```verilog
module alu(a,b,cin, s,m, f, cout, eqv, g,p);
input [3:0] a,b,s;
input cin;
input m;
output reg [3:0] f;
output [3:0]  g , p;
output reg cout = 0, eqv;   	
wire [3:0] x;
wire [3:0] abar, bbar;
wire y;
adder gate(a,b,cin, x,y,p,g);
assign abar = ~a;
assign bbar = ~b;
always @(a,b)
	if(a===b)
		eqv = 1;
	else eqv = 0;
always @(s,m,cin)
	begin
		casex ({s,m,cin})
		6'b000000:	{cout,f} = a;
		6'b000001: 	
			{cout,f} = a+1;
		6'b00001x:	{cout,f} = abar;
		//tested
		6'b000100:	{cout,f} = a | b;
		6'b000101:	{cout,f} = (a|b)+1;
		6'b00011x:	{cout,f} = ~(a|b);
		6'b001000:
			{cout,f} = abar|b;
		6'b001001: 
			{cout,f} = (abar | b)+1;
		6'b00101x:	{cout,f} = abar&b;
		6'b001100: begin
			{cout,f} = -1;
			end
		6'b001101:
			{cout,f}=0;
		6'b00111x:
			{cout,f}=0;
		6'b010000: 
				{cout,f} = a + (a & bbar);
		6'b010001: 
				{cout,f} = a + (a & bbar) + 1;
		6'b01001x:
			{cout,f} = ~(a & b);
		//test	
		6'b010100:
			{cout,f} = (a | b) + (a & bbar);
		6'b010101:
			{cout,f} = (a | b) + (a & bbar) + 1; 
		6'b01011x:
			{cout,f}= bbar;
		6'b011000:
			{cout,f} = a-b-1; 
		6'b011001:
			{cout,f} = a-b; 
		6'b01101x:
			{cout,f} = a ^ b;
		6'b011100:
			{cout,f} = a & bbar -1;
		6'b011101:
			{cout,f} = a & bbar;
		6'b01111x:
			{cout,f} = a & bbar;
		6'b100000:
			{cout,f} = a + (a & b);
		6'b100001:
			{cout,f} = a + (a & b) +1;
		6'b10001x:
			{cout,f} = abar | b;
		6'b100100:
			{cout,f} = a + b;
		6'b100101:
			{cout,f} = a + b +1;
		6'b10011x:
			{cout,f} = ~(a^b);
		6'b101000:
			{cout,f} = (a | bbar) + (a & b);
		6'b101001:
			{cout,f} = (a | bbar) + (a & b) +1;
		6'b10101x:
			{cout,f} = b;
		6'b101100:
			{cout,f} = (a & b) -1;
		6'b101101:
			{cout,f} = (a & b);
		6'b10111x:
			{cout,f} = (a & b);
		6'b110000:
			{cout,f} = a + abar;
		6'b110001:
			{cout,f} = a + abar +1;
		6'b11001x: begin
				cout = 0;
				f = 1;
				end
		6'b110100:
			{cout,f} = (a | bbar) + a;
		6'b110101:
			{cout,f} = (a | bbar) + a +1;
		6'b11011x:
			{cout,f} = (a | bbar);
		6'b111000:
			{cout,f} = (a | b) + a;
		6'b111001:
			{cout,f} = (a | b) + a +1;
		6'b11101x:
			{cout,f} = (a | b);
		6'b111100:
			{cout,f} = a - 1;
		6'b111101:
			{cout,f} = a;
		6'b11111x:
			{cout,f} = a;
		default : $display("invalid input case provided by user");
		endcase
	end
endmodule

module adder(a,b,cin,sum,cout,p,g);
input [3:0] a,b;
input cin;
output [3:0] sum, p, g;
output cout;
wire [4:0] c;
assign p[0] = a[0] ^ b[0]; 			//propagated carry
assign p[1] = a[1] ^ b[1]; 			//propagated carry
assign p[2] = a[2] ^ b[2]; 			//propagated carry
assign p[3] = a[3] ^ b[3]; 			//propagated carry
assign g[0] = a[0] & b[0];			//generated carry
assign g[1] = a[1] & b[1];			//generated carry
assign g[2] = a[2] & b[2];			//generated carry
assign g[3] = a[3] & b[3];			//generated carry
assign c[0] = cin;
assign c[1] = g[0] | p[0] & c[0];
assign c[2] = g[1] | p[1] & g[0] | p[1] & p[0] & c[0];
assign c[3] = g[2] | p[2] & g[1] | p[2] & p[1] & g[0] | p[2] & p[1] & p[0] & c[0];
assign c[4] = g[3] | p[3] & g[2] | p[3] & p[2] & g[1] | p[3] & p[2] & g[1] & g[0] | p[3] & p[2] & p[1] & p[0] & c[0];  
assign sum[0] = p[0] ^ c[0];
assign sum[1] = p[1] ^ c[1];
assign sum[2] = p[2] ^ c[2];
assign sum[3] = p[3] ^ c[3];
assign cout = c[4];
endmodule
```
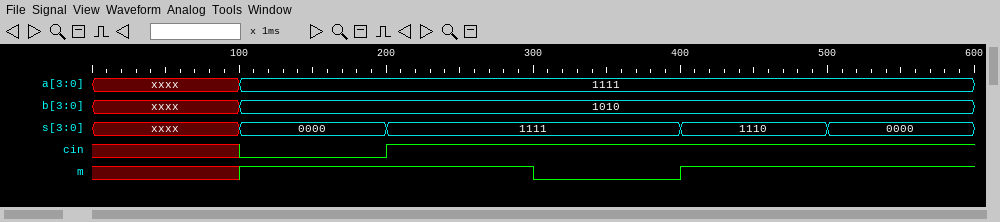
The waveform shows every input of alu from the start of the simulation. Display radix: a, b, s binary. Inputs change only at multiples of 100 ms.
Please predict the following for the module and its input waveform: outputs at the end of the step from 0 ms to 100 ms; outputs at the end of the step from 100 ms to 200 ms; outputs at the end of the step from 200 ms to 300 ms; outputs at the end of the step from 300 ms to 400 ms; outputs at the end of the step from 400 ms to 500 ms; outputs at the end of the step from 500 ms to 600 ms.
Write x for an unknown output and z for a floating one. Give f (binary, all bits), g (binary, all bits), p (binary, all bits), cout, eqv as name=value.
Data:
f=x, g=x, p=x, cout=0, eqv=x
f=0000, g=1010, p=0101, cout=0, eqv=0
f=1111, g=1010, p=0101, cout=0, eqv=0
f=1111, g=1010, p=0101, cout=0, eqv=0
f=1111, g=1010, p=0101, cout=0, eqv=0
f=0000, g=1010, p=0101, cout=0, eqv=0
